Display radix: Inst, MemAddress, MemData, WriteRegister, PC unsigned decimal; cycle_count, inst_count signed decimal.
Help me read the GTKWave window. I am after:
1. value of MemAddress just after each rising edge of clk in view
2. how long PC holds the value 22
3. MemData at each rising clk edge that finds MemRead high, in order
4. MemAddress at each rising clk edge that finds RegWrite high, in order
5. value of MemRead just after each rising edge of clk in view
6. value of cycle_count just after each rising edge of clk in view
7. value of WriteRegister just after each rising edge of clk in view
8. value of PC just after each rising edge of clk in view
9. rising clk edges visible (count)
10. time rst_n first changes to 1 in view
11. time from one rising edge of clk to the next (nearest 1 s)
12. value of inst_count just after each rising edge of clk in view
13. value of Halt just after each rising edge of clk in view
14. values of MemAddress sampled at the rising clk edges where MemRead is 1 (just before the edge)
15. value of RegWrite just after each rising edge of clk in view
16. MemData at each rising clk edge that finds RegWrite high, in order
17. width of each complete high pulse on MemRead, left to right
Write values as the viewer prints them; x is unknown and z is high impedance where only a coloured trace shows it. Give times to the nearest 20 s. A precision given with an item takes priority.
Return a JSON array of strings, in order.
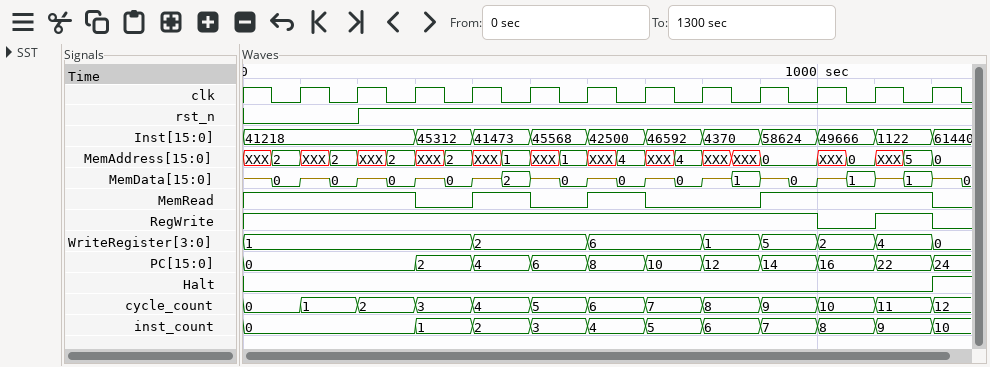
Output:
["XXX, XXX, XXX, XXX, XXX, XXX, XXX, XXX, 0, XXX, XXX, 0", "100 s", "0, 0, 0, 2, 0, 0, 1, 1", "2, 2, 2, 2, 1, 1, 4, 4, XXX, 0, 5", "1 1 0 1 0 1 0 0 1 1 1 0", "1, 2, 3, 4, 5, 6, 7, 8, 9, 10, 11, 12", "1, 1, 1, 2, 2, 6, 6, 1, 5, 2, 4, 0", "0, 0, 2, 4, 6, 8, 10, 12, 14, 16, 22, 24", "12", "200 s", "100 s", "0, 0, 1, 2, 3, 4, 5, 6, 7, 8, 9, 10", "0 0 0 0 0 0 0 0 0 0 0 1", "2, 2, 2, 1, 4, 0, 0, 5", "1 1 1 1 1 1 1 1 1 0 1 0", "0, 0, 0, 0, 2, 0, 0, 0, 1, 0, 1", "100 s, 100 s, 300 s"]
